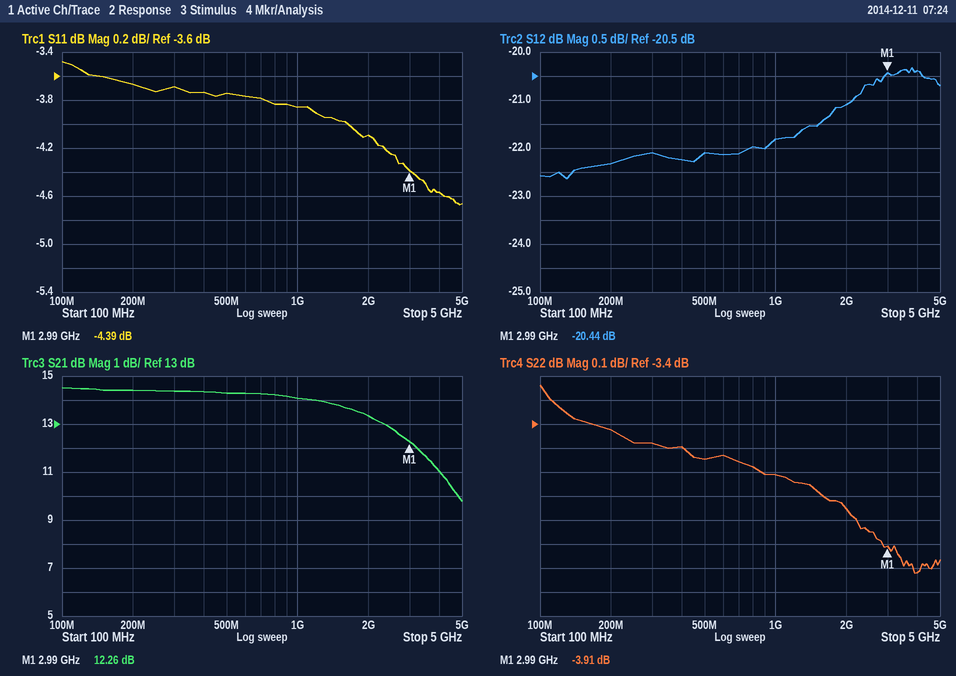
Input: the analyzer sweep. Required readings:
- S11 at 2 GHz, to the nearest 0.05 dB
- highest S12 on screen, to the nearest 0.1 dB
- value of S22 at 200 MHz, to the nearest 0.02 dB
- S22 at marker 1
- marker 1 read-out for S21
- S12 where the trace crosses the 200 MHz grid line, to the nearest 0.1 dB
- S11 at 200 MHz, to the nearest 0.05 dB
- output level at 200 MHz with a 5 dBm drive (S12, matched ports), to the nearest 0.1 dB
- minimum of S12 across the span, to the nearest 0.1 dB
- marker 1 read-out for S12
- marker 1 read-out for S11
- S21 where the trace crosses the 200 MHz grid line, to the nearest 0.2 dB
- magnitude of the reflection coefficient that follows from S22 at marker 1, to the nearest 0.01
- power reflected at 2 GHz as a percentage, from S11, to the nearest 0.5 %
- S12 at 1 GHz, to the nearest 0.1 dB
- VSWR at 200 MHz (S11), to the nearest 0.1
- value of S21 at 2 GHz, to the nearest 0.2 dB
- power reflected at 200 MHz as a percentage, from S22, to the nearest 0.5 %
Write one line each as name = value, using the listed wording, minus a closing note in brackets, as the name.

S11 at 2 GHz, to the nearest 0.05 dB = -4.10 dB
highest S12 on screen, to the nearest 0.1 dB = -20.3 dB
value of S22 at 200 MHz, to the nearest 0.02 dB = -3.42 dB
S22 at marker 1 = -3.91 dB
marker 1 read-out for S21 = 12.26 dB
S12 where the trace crosses the 200 MHz grid line, to the nearest 0.1 dB = -22.3 dB
S11 at 200 MHz, to the nearest 0.05 dB = -3.65 dB
output level at 200 MHz with a 5 dBm drive (S12, matched ports), to the nearest 0.1 dB = -17.3 dBm
minimum of S12 across the span, to the nearest 0.1 dB = -22.6 dB
marker 1 read-out for S12 = -20.44 dB
marker 1 read-out for S11 = -4.39 dB
S21 where the trace crosses the 200 MHz grid line, to the nearest 0.2 dB = 14.4 dB
magnitude of the reflection coefficient that follows from S22 at marker 1, to the nearest 0.01 = 0.64
power reflected at 2 GHz as a percentage, from S11, to the nearest 0.5 % = 39.0 %
S12 at 1 GHz, to the nearest 0.1 dB = -21.8 dB
VSWR at 200 MHz (S11), to the nearest 0.1 = 4.8
value of S21 at 2 GHz, to the nearest 0.2 dB = 13.4 dB
power reflected at 200 MHz as a percentage, from S22, to the nearest 0.5 % = 45.5 %
